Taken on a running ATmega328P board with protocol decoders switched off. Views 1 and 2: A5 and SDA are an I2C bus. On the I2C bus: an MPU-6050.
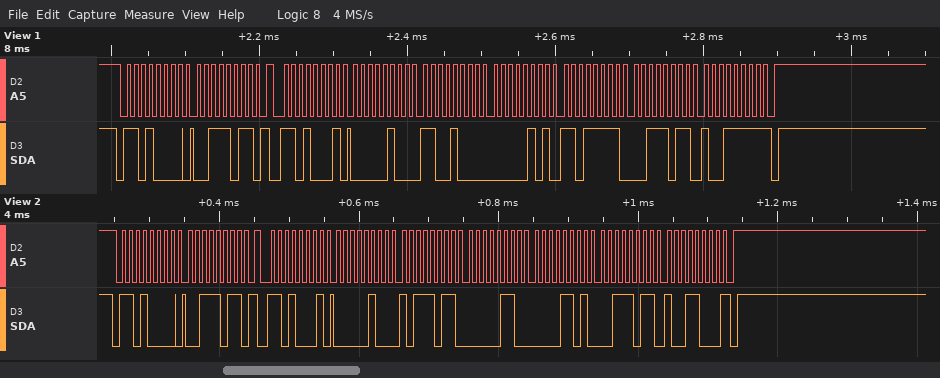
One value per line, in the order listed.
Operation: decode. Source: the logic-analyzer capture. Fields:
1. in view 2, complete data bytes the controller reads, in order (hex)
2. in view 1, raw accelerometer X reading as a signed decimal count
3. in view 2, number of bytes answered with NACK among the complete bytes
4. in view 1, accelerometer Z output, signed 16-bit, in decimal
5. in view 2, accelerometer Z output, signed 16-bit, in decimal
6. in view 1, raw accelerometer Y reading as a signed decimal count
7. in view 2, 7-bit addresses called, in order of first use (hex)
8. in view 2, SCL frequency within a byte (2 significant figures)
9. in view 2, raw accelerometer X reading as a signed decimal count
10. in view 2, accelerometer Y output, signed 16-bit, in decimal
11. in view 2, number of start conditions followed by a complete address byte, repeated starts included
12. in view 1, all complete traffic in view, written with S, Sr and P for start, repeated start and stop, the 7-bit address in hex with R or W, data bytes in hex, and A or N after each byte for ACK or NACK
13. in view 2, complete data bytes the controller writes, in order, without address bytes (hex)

04 BB 06 0D 3B 98
1224
1
15263
15256
1503
0x68
100 kHz
1211
1549
2
S 68W A 3B A Sr 68R A 04 A C8 A 05 A DF A 3B A 9F N P
3B
